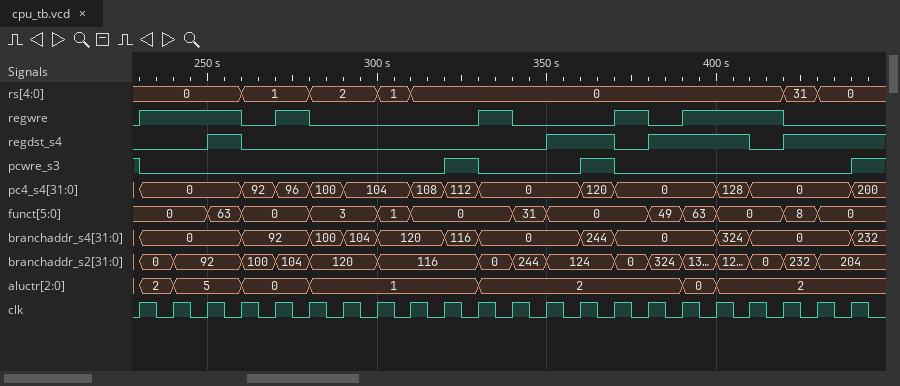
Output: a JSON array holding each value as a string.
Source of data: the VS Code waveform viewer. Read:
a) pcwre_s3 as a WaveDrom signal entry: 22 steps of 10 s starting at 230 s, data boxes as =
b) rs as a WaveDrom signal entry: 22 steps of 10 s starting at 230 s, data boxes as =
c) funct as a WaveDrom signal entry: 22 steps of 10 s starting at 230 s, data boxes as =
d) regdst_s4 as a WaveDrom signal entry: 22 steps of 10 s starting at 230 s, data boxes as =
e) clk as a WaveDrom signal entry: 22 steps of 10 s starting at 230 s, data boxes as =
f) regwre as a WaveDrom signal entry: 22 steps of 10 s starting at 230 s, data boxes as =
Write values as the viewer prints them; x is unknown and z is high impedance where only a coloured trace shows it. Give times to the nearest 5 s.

["{name: 'pcwre_s3', wave: '0........10..10......1'}", "{name: 'rs', wave: '=..=.=.==..........==.', data: '0 1 2 1 0 31 0'}", "{name: 'funct', wave: '=.==.=.==..==..===.==.', data: '0 63 0 3 1 0 31 0 49 63 0 8 0'}", "{name: 'regdst_s4', wave: '0.10........1.01..01..'}", "{name: 'clk', wave: 'p.....................'}", "{name: 'regwre', wave: '1..010....10..101..0..'}"]
